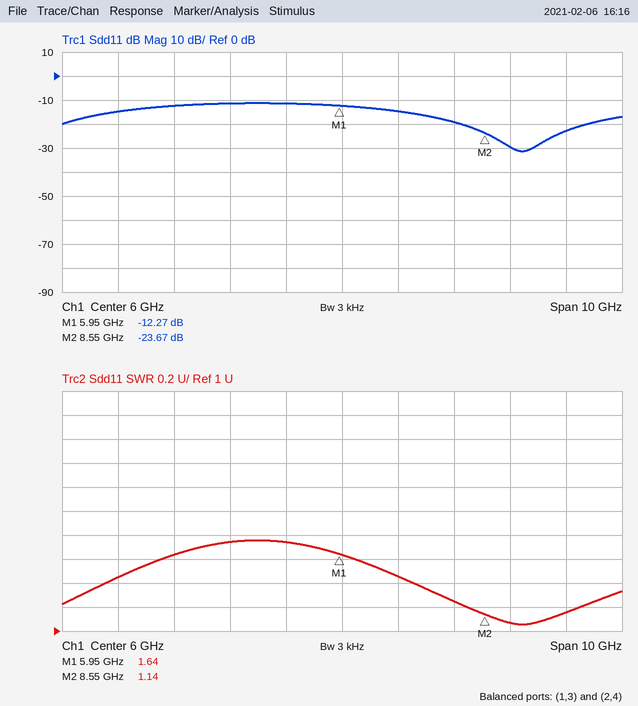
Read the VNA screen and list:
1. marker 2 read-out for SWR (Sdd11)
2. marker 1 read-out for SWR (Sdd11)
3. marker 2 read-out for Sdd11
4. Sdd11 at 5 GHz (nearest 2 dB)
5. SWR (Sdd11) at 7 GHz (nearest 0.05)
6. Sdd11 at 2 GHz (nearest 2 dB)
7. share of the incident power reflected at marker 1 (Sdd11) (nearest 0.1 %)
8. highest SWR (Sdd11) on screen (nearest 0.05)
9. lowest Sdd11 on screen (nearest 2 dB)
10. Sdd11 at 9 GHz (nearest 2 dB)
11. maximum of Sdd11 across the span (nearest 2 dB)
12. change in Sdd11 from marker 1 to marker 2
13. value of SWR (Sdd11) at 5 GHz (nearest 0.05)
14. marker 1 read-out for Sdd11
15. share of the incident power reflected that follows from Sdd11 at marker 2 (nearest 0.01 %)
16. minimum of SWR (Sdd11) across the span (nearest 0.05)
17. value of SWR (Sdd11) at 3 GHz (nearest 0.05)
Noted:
1.14
1.64
-23.67 dB
-12 dB
1.45
-14 dB
5.9 %
1.75
-32 dB
-30 dB
-12 dB
-11.40 dB
1.75
-12.27 dB
0.43 %
1.05
1.65
